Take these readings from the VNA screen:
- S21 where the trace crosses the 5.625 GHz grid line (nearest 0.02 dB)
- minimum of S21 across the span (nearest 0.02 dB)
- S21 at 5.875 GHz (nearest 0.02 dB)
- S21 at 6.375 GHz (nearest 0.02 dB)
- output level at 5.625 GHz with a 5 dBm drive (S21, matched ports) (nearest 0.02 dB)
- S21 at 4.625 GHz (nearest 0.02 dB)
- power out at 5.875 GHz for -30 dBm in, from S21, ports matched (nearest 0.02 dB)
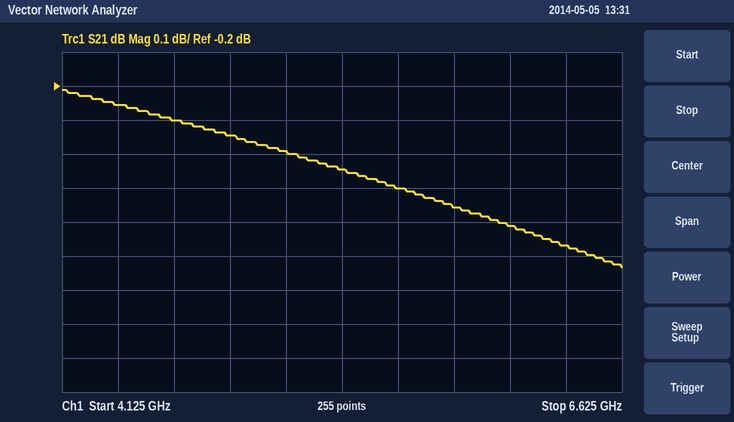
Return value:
-0.50 dB
-0.74 dB
-0.56 dB
-0.66 dB
4.50 dBm
-0.30 dB
-30.56 dBm
